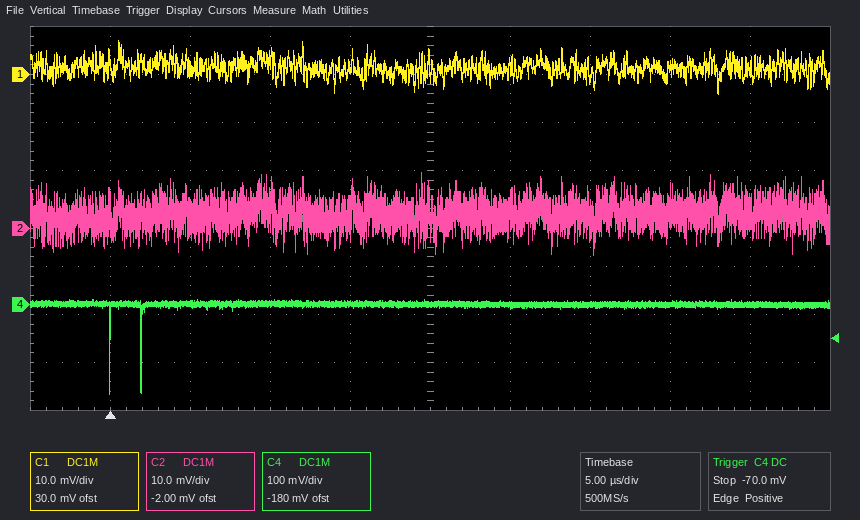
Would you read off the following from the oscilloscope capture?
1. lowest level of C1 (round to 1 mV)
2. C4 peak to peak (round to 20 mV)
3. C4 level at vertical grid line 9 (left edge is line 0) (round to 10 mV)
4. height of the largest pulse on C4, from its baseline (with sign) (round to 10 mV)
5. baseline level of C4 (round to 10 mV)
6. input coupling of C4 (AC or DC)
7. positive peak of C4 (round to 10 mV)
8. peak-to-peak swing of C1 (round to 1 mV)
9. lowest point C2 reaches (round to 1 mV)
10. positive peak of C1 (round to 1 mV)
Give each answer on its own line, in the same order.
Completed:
-4 mV
200 mV
0 mV
-190 mV
0 mV
DC
10 mV
11 mV
-6 mV
7 mV
